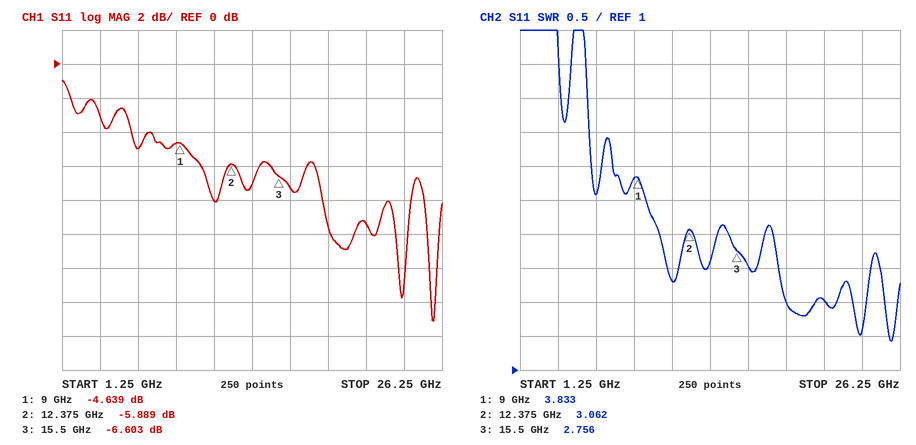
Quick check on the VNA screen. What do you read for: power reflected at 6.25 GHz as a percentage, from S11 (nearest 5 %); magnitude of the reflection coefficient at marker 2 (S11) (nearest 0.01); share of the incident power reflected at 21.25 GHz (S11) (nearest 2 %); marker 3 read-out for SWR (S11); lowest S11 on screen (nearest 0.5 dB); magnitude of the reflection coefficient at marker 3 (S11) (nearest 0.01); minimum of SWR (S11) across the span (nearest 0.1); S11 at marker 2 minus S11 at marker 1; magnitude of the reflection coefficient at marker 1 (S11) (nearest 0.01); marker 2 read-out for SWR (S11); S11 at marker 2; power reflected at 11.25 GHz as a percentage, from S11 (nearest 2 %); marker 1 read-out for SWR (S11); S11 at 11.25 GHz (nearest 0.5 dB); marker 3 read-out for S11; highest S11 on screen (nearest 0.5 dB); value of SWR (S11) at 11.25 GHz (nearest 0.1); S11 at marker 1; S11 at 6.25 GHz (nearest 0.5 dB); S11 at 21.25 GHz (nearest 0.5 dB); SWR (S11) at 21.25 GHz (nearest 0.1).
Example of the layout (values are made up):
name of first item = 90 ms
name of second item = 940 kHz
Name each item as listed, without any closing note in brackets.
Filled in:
power reflected at 6.25 GHz as a percentage, from S11 = 30 %
magnitude of the reflection coefficient at marker 2 (S11) = 0.51
share of the incident power reflected at 21.25 GHz (S11) = 12 %
marker 3 read-out for SWR = 2.756
lowest S11 on screen = -15.0 dB
magnitude of the reflection coefficient at marker 3 (S11) = 0.47
minimum of SWR (S11) across the span = 1.4
S11 at marker 2 minus S11 at marker 1 = -1.250 dB
magnitude of the reflection coefficient at marker 1 (S11) = 0.59
marker 2 read-out for SWR = 3.062
S11 at marker 2 = -5.889 dB
power reflected at 11.25 GHz as a percentage, from S11 = 16 %
marker 1 read-out for SWR = 3.833
S11 at 11.25 GHz = -8.0 dB
marker 3 read-out for S11 = -6.603 dB
highest S11 on screen = -1.0 dB
value of SWR (S11) at 11.25 GHz = 2.3
S11 at marker 1 = -4.639 dB
S11 at 6.25 GHz = -5.0 dB
S11 at 21.25 GHz = -9.5 dB
SWR (S11) at 21.25 GHz = 2.0
